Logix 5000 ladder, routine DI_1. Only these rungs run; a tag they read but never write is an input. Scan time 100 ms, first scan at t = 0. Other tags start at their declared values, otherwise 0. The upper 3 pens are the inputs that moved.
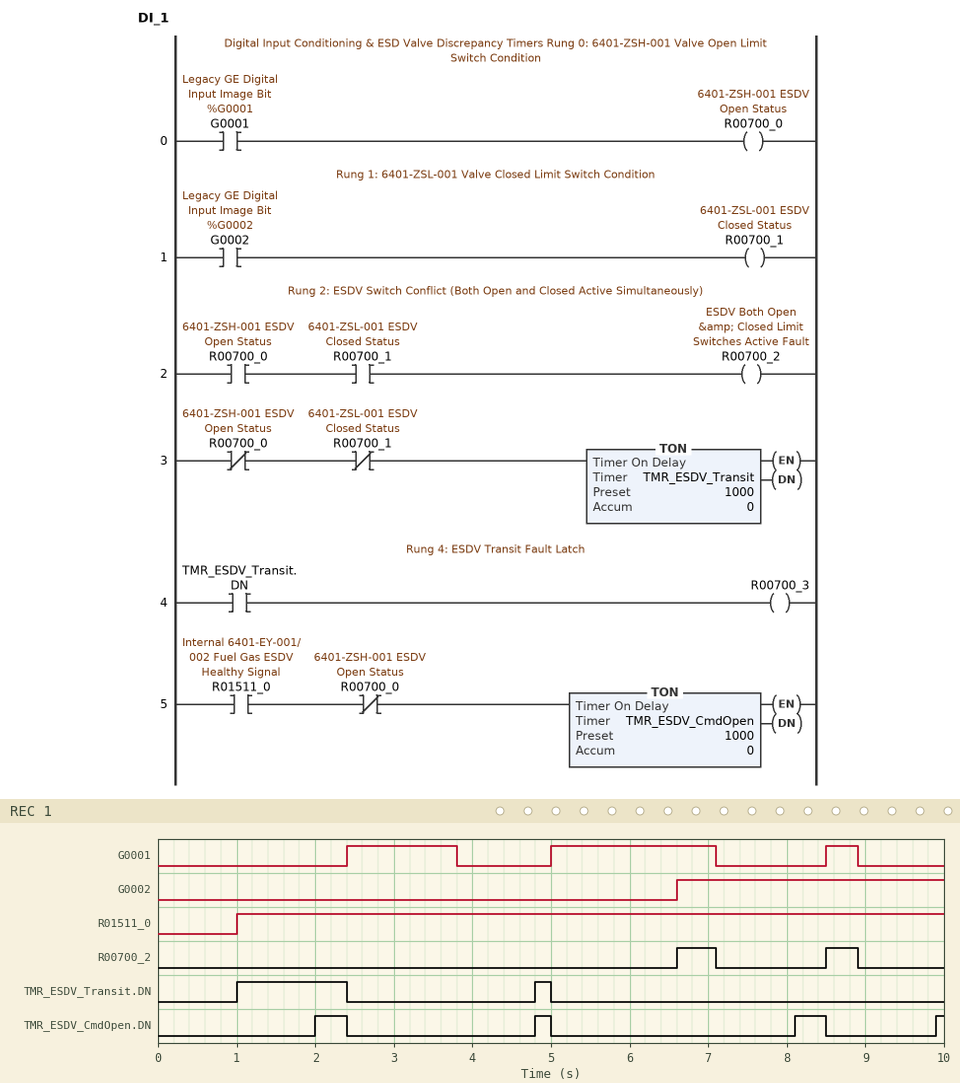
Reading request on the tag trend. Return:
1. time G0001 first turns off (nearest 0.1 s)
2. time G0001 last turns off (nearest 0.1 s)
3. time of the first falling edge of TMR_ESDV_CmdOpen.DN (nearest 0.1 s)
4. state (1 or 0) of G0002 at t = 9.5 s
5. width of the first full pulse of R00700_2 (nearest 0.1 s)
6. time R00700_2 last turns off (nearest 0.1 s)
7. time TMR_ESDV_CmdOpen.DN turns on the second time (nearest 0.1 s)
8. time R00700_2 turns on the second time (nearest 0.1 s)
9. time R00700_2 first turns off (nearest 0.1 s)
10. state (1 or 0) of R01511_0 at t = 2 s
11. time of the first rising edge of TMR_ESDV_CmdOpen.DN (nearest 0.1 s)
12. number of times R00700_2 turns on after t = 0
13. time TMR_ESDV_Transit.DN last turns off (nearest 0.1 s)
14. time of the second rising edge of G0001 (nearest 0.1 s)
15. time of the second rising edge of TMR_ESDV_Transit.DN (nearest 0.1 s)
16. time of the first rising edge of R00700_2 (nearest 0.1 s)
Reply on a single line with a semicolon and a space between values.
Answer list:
3.8 s; 8.9 s; 2.4 s; 1; 0.5 s; 8.9 s; 4.8 s; 8.5 s; 7.1 s; 1; 2.0 s; 2; 5.0 s; 5.0 s; 4.8 s; 6.6 s
